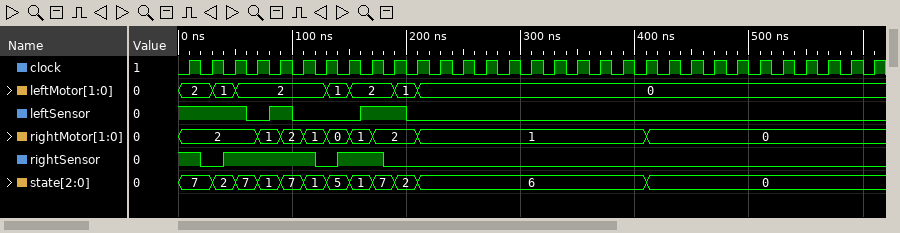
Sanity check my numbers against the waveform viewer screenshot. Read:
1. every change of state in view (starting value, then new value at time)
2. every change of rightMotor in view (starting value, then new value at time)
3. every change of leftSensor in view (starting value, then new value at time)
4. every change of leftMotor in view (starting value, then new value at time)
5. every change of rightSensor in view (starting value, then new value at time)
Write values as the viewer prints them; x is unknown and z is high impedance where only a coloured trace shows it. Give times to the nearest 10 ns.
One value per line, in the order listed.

7, 2 at 30 ns, 7 at 50 ns, 1 at 70 ns, 7 at 90 ns, 1 at 110 ns, 5 at 130 ns, 1 at 150 ns, 7 at 170 ns, 2 at 190 ns, 6 at 210 ns, 0 at 410 ns
2, 1 at 70 ns, 2 at 90 ns, 1 at 110 ns, 0 at 130 ns, 1 at 150 ns, 2 at 170 ns, 1 at 210 ns, 0 at 410 ns
1, 0 at 60 ns, 1 at 80 ns, 0 at 100 ns, 1 at 160 ns, 0 at 200 ns
2, 1 at 30 ns, 2 at 50 ns, 1 at 130 ns, 2 at 150 ns, 1 at 190 ns, 0 at 210 ns
1, 0 at 20 ns, 1 at 40 ns, 0 at 120 ns, 1 at 140 ns, 0 at 180 ns
